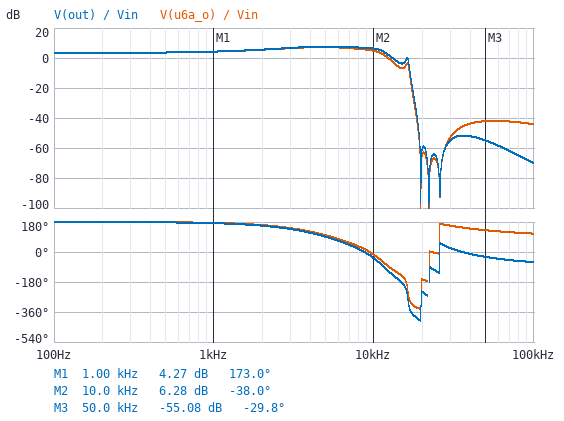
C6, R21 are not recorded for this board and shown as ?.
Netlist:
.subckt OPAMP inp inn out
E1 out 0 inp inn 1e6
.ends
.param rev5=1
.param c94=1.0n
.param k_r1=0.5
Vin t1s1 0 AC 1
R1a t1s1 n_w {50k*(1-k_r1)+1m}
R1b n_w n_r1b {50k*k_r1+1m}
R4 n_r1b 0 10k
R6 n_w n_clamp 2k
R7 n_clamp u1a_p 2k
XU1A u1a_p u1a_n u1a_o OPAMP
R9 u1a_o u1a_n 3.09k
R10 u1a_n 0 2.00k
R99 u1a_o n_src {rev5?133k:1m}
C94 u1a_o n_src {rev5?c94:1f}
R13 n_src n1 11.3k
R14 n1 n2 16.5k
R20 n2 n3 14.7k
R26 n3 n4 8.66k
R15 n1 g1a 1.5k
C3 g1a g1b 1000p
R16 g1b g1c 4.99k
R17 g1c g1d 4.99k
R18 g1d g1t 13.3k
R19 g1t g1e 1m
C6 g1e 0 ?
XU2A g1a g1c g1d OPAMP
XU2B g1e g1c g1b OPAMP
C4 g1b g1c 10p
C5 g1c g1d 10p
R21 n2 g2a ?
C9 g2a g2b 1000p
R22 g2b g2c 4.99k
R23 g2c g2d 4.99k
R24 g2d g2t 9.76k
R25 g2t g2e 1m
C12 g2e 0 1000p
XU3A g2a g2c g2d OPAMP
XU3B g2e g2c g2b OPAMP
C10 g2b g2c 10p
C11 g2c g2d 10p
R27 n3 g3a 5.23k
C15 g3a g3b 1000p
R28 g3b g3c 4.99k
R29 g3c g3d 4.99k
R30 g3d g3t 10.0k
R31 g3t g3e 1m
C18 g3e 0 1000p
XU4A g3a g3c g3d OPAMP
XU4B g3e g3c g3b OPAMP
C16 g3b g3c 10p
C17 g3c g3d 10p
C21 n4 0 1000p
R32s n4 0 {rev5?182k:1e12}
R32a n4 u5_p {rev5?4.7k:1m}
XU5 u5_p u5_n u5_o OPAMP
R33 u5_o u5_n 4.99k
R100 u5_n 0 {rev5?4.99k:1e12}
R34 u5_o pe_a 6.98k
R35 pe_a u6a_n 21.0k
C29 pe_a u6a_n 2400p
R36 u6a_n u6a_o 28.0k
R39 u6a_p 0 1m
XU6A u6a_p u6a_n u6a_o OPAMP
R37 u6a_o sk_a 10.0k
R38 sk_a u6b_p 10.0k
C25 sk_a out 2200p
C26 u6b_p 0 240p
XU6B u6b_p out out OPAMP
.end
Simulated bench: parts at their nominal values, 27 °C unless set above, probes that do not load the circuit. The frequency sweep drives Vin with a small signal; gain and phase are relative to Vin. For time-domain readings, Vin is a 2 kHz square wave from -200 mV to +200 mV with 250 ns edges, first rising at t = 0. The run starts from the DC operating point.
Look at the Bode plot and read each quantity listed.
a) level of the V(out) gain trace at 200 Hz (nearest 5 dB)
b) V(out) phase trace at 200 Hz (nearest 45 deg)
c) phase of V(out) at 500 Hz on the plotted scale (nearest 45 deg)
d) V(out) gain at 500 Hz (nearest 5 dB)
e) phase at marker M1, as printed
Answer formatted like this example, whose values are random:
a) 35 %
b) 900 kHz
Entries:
a) 5 dB
b) 180 deg
c) 180 deg
d) 5 dB
e) 173.0 deg
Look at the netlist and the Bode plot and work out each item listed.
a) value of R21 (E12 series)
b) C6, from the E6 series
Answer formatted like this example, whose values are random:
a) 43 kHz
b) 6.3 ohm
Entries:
a) 3.9 kΩ
b) 3.3 nF
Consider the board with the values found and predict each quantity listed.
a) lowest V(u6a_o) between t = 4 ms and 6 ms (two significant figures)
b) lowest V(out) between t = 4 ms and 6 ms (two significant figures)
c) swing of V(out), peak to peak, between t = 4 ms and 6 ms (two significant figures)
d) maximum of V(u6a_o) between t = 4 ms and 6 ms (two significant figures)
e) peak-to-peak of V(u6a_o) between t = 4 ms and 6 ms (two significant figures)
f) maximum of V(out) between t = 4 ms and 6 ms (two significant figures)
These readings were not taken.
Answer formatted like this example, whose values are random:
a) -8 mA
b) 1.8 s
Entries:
a) -620 mV
b) -660 mV
c) 1.3 V
d) 620 mV
e) 1.2 V
f) 660 mV
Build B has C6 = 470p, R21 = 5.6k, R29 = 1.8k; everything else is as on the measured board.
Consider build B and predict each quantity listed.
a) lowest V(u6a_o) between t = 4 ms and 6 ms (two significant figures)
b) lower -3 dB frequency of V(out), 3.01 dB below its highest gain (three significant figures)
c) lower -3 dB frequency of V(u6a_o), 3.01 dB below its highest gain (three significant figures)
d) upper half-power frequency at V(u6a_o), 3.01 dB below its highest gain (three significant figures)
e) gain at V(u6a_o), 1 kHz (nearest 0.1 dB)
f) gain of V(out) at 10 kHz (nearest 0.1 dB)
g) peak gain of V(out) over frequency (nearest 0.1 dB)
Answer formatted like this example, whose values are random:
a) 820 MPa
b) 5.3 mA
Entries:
a) -580 mV
b) 2.03 kHz
c) 1.71 kHz
d) 8.94 kHz
e) 3.9 dB
f) 4.7 dB
g) 8.1 dB
